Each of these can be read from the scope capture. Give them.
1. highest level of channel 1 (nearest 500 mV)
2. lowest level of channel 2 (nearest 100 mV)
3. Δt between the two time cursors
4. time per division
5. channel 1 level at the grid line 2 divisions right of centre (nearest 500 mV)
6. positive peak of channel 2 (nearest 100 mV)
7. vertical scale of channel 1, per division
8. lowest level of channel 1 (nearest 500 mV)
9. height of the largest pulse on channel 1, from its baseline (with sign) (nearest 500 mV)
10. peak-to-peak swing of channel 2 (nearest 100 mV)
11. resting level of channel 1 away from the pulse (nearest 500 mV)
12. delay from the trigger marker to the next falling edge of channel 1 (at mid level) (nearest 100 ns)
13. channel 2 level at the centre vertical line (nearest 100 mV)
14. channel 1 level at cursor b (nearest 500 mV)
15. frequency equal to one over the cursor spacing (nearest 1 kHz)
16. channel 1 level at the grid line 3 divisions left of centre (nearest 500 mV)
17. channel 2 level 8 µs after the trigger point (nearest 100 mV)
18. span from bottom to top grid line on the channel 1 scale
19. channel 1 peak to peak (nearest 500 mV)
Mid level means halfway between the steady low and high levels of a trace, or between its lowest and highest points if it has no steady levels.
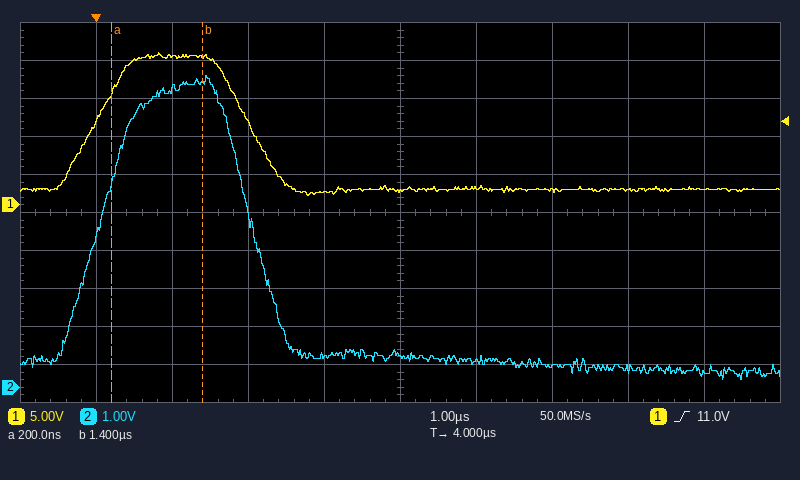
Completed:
20.0 V
200 mV
1.2 µs
1 µs
2.0 V
8.2 V
5 V
1.0 V
+18.0 V
8.0 V
2.0 V
2.0 µs
800 mV
19.5 V
833 kHz
19.5 V
400 mV
50 V
19.0 V
